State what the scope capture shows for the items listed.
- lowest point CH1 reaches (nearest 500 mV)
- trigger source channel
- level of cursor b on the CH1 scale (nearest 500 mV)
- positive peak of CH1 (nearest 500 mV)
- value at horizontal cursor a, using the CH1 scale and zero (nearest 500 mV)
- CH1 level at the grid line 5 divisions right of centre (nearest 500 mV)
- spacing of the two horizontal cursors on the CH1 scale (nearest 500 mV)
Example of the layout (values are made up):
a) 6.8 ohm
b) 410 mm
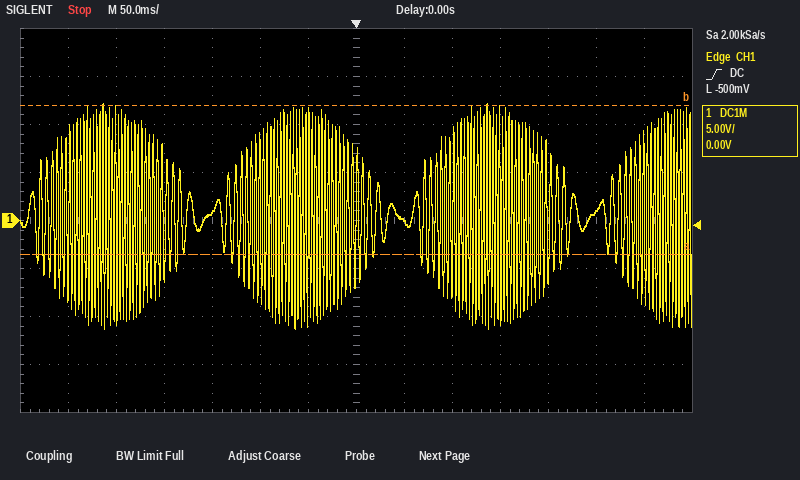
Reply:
a) -11.0 V
b) CH1
c) 12.0 V
d) 12.0 V
e) -3.5 V
f) 1.0 V
g) 15.5 V
